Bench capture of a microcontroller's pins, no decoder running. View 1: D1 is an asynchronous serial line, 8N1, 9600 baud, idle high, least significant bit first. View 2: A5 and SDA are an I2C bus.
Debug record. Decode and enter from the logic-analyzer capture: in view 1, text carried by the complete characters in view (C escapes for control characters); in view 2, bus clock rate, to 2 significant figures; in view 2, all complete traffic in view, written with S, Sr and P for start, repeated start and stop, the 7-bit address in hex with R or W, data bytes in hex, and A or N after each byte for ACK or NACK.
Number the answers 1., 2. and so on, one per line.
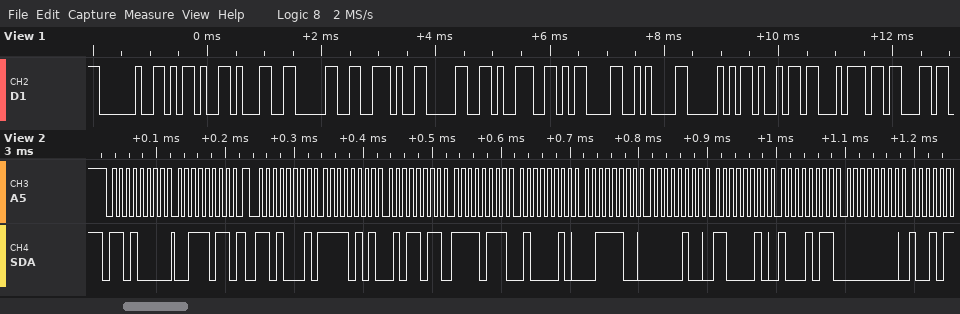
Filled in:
1. " -10.09\r\nPitc"
2. 100 kHz
3. S 68W A 3B A Sr 68R A F5 A 5B A F7 A 42 A 3C A 04 A C2 A 8B A 00 A
